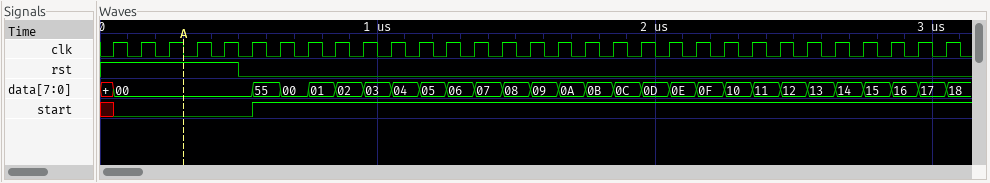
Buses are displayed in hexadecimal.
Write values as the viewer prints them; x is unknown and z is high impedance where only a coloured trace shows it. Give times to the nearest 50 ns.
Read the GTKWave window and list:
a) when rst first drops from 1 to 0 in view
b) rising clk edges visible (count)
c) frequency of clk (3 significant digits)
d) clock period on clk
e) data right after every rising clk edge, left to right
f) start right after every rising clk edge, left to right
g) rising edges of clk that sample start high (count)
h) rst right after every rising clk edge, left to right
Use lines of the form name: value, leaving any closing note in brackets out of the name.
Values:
when rst first drops from 1 to 0 in view: 500 ns
rising clk edges visible: 31
frequency of clk: 10.0 MHz
clock period on clk: 100 ns
data right after every rising clk edge, left to right: 00, 00, 00, 00, 00, 55, 00, 01, 02, 03, 04, 05, 06, 07, 08, 09, 0A, 0B, 0C, 0D, 0E, 0F, 10, 11, 12, 13, 14, 15, 16, 17, 18
start right after every rising clk edge, left to right: 0 0 0 0 0 1 1 1 1 1 1 1 1 1 1 1 1 1 1 1 1 1 1 1 1 1 1 1 1 1 1
rising edges of clk that sample start high: 25
rst right after every rising clk edge, left to right: 1 1 1 1 1 0 0 0 0 0 0 0 0 0 0 0 0 0 0 0 0 0 0 0 0 0 0 0 0 0 0
